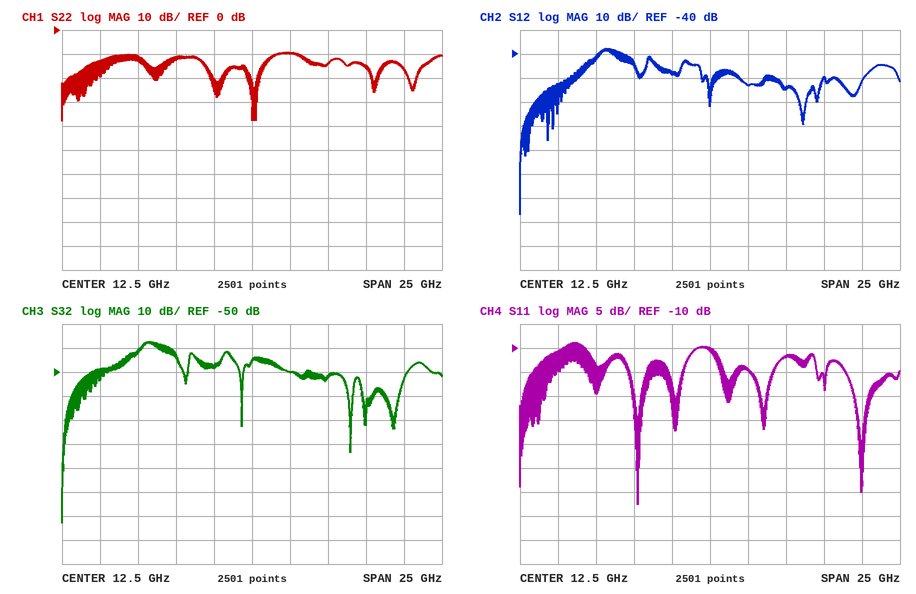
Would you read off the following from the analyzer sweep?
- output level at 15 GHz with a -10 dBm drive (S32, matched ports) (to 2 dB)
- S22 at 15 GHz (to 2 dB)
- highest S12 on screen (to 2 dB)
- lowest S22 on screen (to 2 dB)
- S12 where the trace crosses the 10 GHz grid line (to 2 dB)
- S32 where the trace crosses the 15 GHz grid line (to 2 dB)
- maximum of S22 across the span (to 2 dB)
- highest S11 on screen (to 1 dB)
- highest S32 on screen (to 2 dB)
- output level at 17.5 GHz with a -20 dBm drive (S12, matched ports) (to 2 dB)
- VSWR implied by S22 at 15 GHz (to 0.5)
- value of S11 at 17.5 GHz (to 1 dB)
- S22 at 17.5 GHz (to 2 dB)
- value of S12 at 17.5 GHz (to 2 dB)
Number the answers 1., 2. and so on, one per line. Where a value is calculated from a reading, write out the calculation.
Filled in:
1. -10 dBm + (-50 dB) = -60 dBm
2. -10 dB
3. -38 dB
4. -38 dB
5. -48 dB
6. -50 dB
7. -10 dB
8. -9 dB
9. -38 dB
10. -20 dBm + (-54 dB) = -74 dBm
11. |Γ| = 10^(-10/20) = 0.3162; VSWR = (1 + 0.3162)/(1 − 0.3162) ≈ 1.92, so 2.0 to the nearest 0.5
12. -12 dB
13. -14 dB
14. -54 dB
